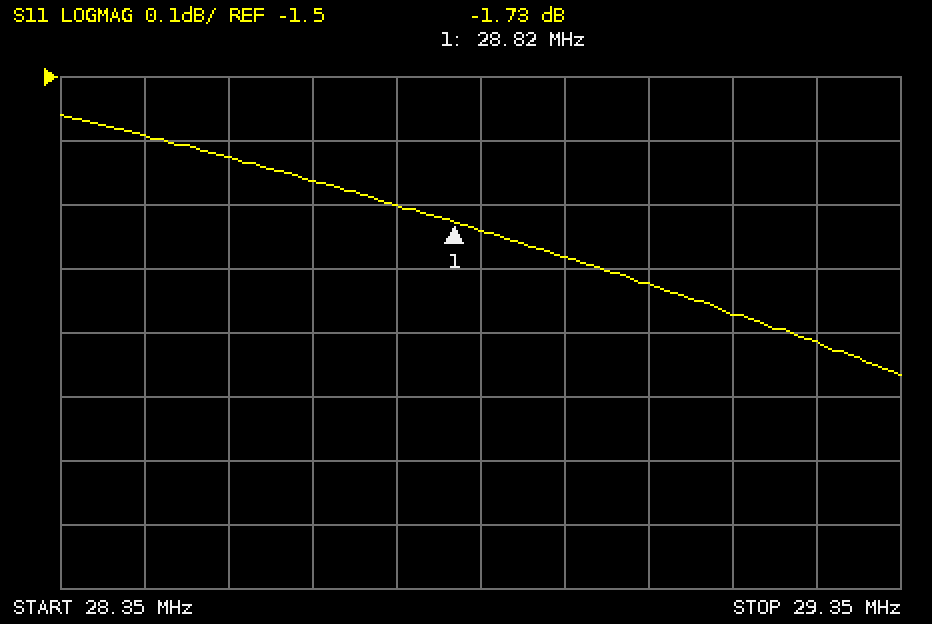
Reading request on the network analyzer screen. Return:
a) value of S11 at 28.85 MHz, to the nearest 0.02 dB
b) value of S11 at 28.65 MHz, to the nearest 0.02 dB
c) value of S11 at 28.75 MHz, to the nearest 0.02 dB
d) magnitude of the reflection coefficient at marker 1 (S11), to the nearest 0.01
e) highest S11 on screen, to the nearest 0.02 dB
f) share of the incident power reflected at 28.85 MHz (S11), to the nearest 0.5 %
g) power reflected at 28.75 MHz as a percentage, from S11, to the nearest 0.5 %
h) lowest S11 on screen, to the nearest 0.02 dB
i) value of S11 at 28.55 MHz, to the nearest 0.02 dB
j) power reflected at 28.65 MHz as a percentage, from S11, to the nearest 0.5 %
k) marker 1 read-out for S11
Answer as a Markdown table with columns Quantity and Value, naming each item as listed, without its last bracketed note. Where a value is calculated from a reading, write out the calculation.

| Quantity | Value |
|---|---|
| value of S11 at 28.85 MHz, to the nearest 0.02 dB | -1.74 dB |
| value of S11 at 28.65 MHz, to the nearest 0.02 dB | -1.66 dB |
| value of S11 at 28.75 MHz, to the nearest 0.02 dB | -1.70 dB |
| magnitude of the reflection coefficient at marker 1 (S11), to the nearest 0.01 | 10^(-1.73/20) ≈ 0.82 |
| highest S11 on screen, to the nearest 0.02 dB | -1.56 dB |
| share of the incident power reflected at 28.85 MHz (S11), to the nearest 0.5 % | 10^(-1.74/10) ≈ 67.0 % |
| power reflected at 28.75 MHz as a percentage, from S11, to the nearest 0.5 % | 10^(-1.7/10) ≈ 67.6 %, so 67.5 % to the nearest 0.5 % |
| lowest S11 on screen, to the nearest 0.02 dB | -1.96 dB |
| value of S11 at 28.55 MHz, to the nearest 0.02 dB | -1.62 dB |
| power reflected at 28.65 MHz as a percentage, from S11, to the nearest 0.5 % | 10^(-1.66/10) ≈ 68.2 %, so 68.0 % to the nearest 0.5 % |
| marker 1 read-out for S11 | -1.73 dB |
